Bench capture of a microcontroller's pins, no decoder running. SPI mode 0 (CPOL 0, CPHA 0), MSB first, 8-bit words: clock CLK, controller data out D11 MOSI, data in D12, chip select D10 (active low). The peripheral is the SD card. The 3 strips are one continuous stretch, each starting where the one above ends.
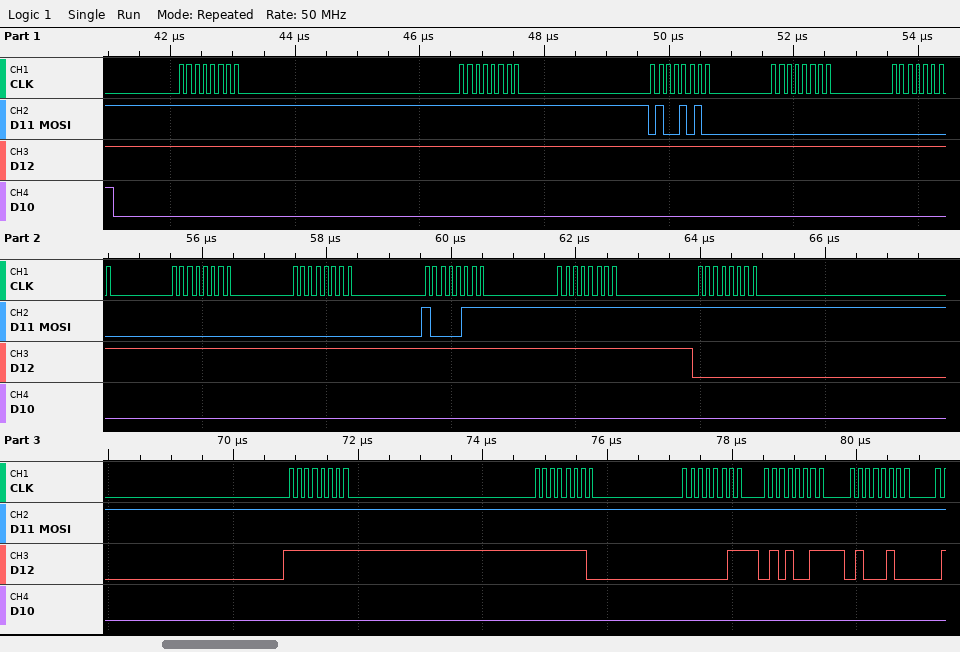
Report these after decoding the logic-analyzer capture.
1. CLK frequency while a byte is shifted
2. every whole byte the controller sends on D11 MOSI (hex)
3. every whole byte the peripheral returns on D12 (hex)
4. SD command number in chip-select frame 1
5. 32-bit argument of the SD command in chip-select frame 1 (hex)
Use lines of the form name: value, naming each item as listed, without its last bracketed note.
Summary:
CLK frequency while a byte is shifted: 8 MHz
every whole byte the controller sends on D11 MOSI: FF FF 4A 00 00 00 00 87 FF FF FF FF FF FF FF
every whole byte the peripheral returns on D12: FF FF FF FF FF FF FF FF FF 00 FF FE 03 53 44
SD command number in chip-select frame 1: CMD10
32-bit argument of the SD command in chip-select frame 1: 0x00000000
